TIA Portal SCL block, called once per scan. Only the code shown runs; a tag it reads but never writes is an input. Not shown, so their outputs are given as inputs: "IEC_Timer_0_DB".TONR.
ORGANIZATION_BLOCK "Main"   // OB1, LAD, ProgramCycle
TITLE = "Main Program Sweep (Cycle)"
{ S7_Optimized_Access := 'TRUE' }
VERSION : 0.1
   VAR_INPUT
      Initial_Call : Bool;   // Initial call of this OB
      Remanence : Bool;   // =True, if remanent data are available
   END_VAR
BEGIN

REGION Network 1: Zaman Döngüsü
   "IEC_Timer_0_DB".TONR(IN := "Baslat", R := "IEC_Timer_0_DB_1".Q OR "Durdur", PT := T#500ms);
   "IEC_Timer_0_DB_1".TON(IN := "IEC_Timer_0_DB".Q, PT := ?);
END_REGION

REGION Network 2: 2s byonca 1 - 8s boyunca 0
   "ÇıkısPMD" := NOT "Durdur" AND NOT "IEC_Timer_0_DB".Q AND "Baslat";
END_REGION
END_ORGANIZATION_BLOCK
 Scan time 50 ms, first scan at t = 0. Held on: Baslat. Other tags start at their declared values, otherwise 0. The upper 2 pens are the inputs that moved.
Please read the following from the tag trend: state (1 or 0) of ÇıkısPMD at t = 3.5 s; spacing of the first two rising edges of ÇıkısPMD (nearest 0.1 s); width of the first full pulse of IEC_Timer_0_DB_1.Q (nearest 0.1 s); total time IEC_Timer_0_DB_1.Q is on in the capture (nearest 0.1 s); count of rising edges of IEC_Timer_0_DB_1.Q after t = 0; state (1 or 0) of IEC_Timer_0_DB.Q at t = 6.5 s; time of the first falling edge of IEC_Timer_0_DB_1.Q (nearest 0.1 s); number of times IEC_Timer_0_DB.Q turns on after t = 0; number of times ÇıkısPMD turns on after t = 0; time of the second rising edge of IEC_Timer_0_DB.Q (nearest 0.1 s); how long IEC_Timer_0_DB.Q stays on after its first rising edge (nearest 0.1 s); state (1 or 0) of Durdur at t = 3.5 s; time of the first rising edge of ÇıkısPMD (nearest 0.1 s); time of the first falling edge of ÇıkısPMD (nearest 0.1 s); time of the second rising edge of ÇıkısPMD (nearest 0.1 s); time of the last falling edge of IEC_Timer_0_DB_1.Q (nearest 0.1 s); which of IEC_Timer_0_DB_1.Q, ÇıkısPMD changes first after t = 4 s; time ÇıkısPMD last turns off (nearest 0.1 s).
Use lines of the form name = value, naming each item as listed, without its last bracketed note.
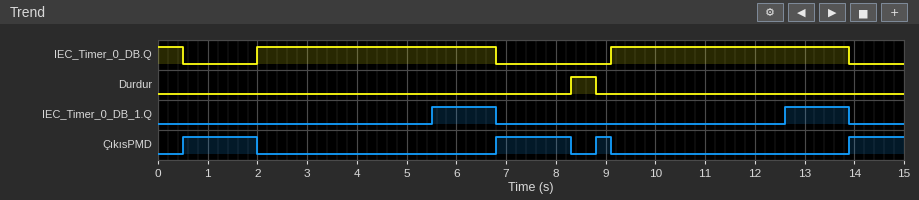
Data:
state (1 or 0) of ÇıkısPMD at t = 3.5 s = 0
spacing of the first two rising edges of ÇıkısPMD = 6.3 s
width of the first full pulse of IEC_Timer_0_DB_1.Q = 1.3 s
total time IEC_Timer_0_DB_1.Q is on in the capture = 2.6 s
count of rising edges of IEC_Timer_0_DB_1.Q after t = 0 = 2
state (1 or 0) of IEC_Timer_0_DB.Q at t = 6.5 s = 1
time of the first falling edge of IEC_Timer_0_DB_1.Q = 6.8 s
number of times IEC_Timer_0_DB.Q turns on after t = 0 = 2
number of times ÇıkısPMD turns on after t = 0 = 4
time of the second rising edge of IEC_Timer_0_DB.Q = 9.1 s
how long IEC_Timer_0_DB.Q stays on after its first rising edge = 4.8 s
state (1 or 0) of Durdur at t = 3.5 s = 0
time of the first rising edge of ÇıkısPMD = 0.5 s
time of the first falling edge of ÇıkısPMD = 2.0 s
time of the second rising edge of ÇıkısPMD = 6.8 s
time of the last falling edge of IEC_Timer_0_DB_1.Q = 13.9 s
which of IEC_Timer_0_DB_1.Q, ÇıkısPMD changes first after t = 4 s = IEC_Timer_0_DB_1.Q
time ÇıkısPMD last turns off = 9.1 s
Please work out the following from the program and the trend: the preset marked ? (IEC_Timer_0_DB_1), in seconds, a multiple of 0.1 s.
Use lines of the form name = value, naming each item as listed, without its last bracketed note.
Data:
the preset marked ? (IEC_Timer_0_DB_1), in seconds, a multiple of 0.1 s = 3.5 s
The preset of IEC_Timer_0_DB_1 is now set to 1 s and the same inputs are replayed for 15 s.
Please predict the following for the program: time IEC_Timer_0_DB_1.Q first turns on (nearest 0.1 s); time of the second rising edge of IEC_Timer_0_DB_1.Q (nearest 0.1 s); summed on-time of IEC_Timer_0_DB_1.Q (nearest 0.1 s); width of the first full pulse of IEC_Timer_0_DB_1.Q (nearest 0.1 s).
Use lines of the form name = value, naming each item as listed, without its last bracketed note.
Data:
time IEC_Timer_0_DB_1.Q first turns on = 3.0 s
time of the second rising edge of IEC_Timer_0_DB_1.Q = 10.1 s
summed on-time of IEC_Timer_0_DB_1.Q = 7.6 s
width of the first full pulse of IEC_Timer_0_DB_1.Q = 3.8 s
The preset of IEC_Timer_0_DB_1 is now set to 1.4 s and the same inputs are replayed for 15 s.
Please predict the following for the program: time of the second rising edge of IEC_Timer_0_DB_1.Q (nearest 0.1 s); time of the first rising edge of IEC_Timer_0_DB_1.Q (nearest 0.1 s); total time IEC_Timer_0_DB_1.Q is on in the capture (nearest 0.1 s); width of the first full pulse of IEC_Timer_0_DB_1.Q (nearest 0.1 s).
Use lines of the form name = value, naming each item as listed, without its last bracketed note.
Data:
time of the second rising edge of IEC_Timer_0_DB_1.Q = 10.5 s
time of the first rising edge of IEC_Timer_0_DB_1.Q = 3.4 s
total time IEC_Timer_0_DB_1.Q is on in the capture = 6.8 s
width of the first full pulse of IEC_Timer_0_DB_1.Q = 3.4 s
